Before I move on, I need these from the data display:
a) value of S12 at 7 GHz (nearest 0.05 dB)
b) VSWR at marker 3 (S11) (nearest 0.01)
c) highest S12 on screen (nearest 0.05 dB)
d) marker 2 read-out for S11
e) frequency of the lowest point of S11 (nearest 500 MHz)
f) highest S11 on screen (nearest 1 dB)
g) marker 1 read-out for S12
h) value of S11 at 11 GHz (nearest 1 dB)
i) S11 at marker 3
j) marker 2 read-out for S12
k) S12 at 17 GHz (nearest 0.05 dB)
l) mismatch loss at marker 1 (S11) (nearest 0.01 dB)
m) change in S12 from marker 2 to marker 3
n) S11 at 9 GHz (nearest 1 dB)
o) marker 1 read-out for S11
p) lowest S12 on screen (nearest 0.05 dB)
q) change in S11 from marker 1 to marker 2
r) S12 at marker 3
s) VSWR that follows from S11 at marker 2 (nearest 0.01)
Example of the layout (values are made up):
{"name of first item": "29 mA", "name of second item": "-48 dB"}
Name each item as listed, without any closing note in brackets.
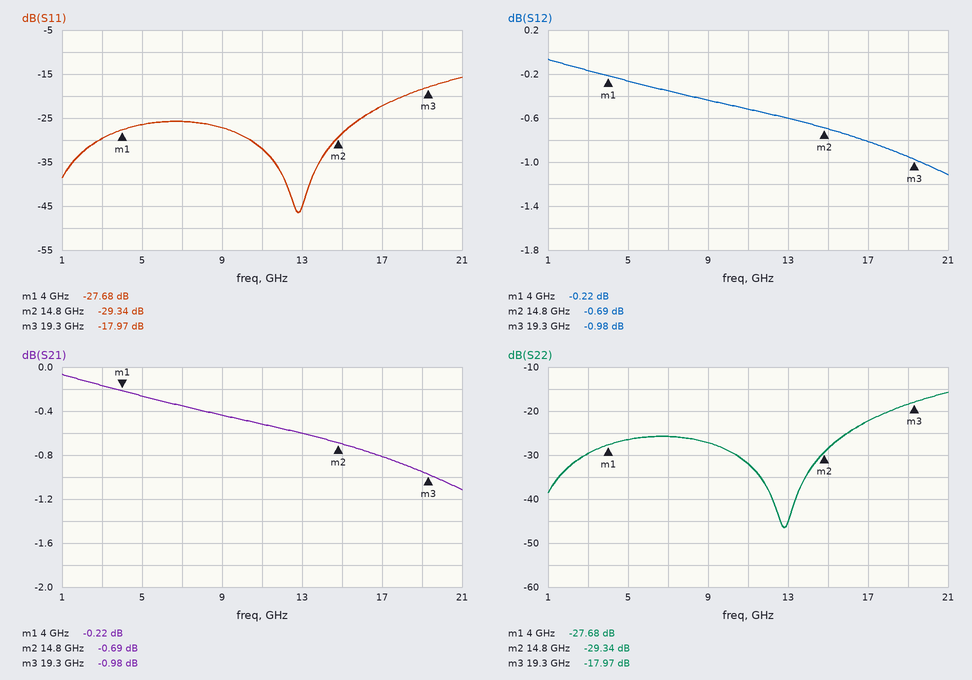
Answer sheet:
{"value of S12 at 7 GHz": "-0.35 dB", "VSWR at marker 3 (S11)": "1.29", "highest S12 on screen": "-0.05 dB", "marker 2 read-out for S11": "-29.34 dB", "frequency of the lowest point of S11": "13.0 GHz", "highest S11 on screen": "-16 dB", "marker 1 read-out for S12": "-0.22 dB", "value of S11 at 11 GHz": "-32 dB", "S11 at marker 3": "-17.97 dB", "marker 2 read-out for S12": "-0.69 dB", "S12 at 17 GHz": "-0.80 dB", "mismatch loss at marker 1 (S11)": "0.01 dB", "change in S12 from marker 2 to marker 3": "-0.29 dB", "S11 at 9 GHz": "-27 dB", "marker 1 read-out for S11": "-27.68 dB", "lowest S12 on screen": "-1.10 dB", "change in S11 from marker 1 to marker 2": "-1.66 dB", "S12 at marker 3": "-0.98 dB", "VSWR that follows from S11 at marker 2": "1.07"}
